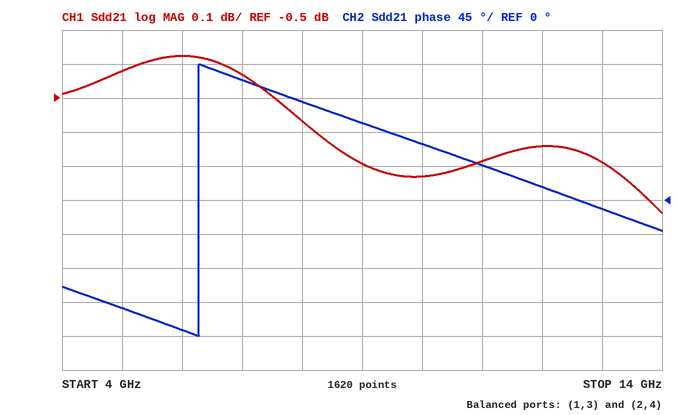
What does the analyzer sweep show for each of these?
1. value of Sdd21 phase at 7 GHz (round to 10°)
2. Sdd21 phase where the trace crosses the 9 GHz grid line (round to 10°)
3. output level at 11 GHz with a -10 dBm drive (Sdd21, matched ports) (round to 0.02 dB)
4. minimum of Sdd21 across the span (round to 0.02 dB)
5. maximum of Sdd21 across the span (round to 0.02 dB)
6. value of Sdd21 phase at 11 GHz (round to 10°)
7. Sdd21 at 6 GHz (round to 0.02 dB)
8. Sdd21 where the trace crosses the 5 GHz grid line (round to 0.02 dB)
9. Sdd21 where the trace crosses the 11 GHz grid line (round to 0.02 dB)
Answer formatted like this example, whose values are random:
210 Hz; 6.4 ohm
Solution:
160°; 100°; -10.68 dBm; -0.84 dB; -0.38 dB; 50°; -0.38 dB; -0.42 dB; -0.68 dB
